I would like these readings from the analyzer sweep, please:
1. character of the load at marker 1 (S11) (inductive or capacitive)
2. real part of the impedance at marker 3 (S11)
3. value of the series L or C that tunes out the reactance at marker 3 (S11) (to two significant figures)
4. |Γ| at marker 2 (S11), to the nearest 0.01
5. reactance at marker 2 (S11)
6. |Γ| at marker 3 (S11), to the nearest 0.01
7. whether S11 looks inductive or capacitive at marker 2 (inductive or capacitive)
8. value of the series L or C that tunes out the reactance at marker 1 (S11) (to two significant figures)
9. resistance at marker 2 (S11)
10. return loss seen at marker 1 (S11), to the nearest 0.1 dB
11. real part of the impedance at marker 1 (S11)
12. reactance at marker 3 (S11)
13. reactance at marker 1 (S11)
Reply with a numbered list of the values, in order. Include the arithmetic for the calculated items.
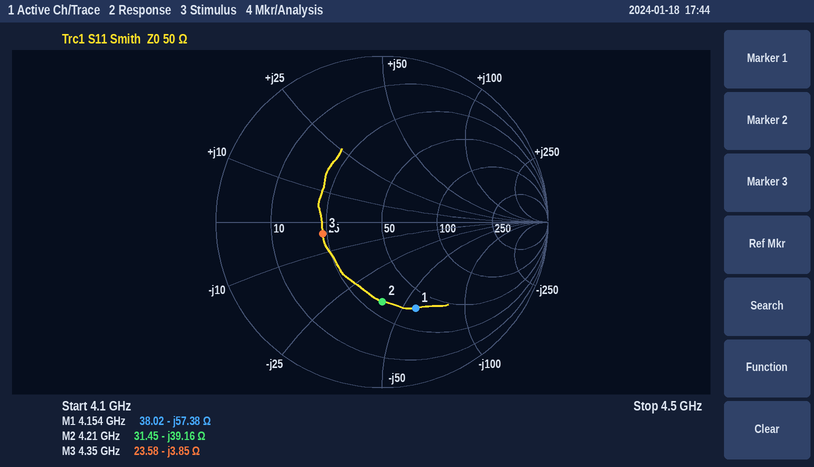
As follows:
1. capacitive
2. 23.58 Ω
3. L = 3.85 Ω/(2π × 4.35 GHz) ≈ 141 pH, so 140 pH to two significant figures
4. 0.48
5. -39.16 Ω
6. 0.36
7. capacitive
8. L = 57.38 Ω/(2π × 4.154 GHz) ≈ 2.2 nH
9. 31.45 Ω
10. 5.1 dB
11. 38.02 Ω
12. -3.85 Ω
13. -57.38 Ω
